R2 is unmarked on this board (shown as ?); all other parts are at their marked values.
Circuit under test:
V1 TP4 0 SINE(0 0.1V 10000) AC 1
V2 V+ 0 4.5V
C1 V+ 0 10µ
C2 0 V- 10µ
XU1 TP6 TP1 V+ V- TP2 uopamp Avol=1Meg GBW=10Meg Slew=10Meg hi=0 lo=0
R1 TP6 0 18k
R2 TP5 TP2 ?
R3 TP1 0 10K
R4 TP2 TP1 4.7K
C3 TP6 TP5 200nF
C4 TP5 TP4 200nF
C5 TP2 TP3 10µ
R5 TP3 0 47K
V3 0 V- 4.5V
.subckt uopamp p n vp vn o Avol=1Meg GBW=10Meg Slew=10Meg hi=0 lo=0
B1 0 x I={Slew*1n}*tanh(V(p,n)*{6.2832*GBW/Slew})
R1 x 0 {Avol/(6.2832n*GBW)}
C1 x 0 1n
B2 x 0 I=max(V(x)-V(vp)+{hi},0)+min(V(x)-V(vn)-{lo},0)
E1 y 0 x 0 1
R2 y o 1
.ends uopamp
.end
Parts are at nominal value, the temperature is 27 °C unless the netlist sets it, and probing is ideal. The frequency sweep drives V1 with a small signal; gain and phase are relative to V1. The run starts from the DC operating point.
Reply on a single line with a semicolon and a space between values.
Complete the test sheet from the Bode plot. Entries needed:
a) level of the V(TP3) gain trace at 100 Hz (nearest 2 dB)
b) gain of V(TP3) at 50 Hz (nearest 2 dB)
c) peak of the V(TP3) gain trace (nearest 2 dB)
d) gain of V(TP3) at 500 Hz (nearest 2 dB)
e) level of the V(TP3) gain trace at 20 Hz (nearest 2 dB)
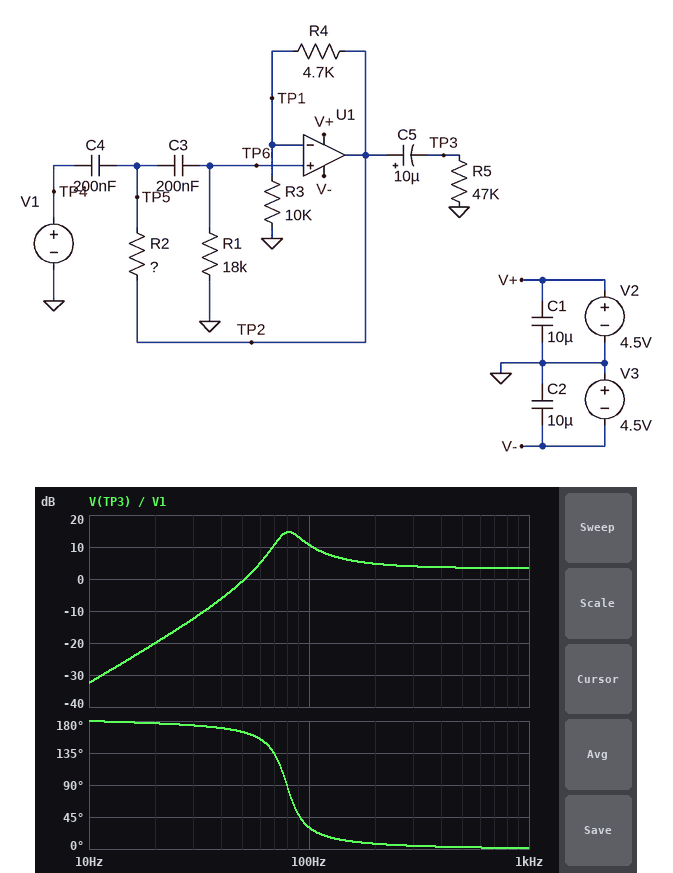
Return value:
10 dB; 0 dB; 14 dB; 4 dB; -20 dB
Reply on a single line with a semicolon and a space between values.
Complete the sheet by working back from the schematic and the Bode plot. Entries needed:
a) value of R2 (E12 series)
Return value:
5.6 kΩ
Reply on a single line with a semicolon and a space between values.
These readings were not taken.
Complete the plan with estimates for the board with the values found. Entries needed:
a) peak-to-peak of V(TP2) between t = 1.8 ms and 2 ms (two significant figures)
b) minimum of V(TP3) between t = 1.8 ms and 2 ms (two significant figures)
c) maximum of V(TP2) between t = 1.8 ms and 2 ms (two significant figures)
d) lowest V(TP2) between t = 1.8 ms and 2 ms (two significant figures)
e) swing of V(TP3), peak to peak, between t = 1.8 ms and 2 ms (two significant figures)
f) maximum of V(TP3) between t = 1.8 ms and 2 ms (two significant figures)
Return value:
290 mV; -150 mV; 150 mV; -150 mV; 290 mV; 150 mV
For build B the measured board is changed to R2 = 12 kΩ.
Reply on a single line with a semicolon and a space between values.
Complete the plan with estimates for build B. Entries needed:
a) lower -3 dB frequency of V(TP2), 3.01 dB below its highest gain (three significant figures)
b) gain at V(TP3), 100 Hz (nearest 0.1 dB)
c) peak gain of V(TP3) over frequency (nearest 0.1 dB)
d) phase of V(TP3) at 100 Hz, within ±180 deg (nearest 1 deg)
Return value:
46.8 Hz; 4.2 dB; 4.3 dB; 39 deg
